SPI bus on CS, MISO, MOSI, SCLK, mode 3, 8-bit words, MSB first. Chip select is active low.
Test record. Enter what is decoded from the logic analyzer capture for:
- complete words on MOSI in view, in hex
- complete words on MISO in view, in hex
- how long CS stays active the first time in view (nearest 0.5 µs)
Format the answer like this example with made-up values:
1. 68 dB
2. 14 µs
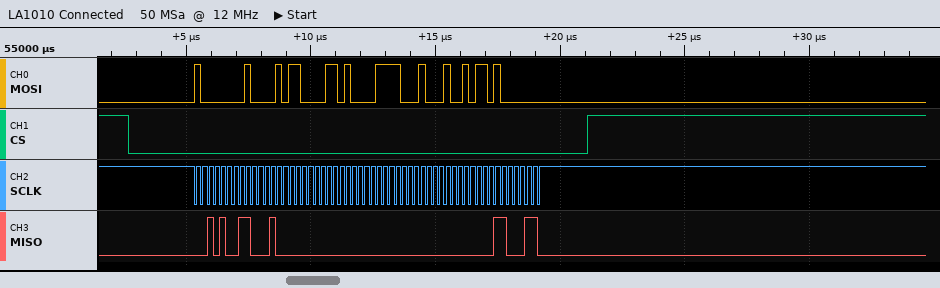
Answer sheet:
1. 80, 85, 86, 87, 88, 96, 80
2. 29, 88, 00, 00, 00, 00, C6
3. 18.5 µs
